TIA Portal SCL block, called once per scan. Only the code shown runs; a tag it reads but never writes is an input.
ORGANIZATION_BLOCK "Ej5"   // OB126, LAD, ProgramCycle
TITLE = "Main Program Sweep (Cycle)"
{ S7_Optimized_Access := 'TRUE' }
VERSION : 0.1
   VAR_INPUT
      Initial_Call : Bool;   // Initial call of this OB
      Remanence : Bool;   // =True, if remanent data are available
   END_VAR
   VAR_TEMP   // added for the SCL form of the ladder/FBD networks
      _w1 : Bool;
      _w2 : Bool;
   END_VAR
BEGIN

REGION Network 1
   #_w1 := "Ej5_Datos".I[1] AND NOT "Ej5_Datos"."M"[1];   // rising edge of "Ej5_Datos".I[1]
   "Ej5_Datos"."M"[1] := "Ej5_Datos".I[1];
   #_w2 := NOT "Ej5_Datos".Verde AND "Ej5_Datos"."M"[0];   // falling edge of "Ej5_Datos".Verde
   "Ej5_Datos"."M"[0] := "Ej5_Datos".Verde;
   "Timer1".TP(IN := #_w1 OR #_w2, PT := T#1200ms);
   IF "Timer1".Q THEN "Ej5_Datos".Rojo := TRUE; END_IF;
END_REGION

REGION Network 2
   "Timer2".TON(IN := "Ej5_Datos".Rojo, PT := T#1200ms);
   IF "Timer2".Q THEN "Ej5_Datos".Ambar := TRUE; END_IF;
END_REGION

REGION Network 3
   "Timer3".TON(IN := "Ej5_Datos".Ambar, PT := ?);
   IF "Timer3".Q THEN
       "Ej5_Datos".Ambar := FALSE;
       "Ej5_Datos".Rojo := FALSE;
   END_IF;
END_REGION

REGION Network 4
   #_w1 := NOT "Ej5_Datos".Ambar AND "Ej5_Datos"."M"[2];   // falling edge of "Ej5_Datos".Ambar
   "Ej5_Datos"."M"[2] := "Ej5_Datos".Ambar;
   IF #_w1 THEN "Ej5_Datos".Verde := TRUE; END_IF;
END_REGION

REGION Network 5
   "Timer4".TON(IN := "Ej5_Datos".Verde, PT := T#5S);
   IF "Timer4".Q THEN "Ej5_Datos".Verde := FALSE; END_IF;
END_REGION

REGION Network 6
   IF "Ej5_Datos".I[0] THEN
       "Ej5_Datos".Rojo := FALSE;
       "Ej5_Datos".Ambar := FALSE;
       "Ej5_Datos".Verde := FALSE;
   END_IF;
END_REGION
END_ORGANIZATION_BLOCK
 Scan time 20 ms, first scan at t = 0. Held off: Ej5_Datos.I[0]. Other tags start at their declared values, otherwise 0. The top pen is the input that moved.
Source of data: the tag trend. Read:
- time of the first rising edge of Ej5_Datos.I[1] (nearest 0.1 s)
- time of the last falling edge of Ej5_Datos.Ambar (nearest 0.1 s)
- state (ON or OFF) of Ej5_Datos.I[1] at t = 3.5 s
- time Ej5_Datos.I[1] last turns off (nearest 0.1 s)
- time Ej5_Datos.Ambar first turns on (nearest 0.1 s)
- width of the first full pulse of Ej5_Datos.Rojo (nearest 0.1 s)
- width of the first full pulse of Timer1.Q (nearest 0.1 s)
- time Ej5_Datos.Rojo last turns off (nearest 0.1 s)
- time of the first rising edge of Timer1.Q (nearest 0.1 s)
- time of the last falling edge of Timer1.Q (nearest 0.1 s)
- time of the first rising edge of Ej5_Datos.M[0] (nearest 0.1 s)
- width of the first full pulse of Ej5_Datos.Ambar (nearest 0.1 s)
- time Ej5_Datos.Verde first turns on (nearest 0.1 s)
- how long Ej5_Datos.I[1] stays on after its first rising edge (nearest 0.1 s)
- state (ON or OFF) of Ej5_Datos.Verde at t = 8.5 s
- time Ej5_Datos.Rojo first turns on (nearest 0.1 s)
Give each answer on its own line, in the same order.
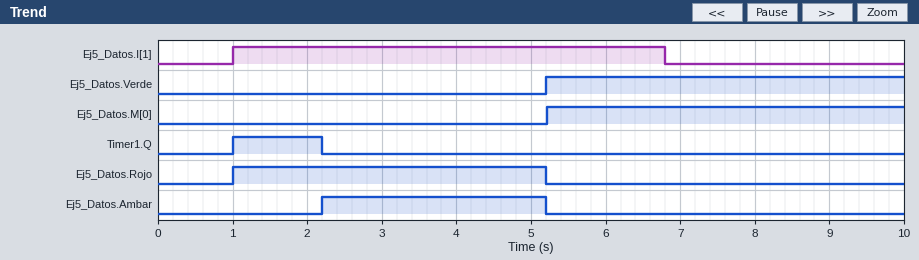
1.0 s
5.2 s
ON
6.8 s
2.2 s
4.2 s
1.2 s
5.2 s
1.0 s
2.2 s
5.2 s
3.0 s
5.2 s
5.8 s
ON
1.0 s
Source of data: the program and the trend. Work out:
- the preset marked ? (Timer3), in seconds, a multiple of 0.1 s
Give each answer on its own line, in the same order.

3.0 s
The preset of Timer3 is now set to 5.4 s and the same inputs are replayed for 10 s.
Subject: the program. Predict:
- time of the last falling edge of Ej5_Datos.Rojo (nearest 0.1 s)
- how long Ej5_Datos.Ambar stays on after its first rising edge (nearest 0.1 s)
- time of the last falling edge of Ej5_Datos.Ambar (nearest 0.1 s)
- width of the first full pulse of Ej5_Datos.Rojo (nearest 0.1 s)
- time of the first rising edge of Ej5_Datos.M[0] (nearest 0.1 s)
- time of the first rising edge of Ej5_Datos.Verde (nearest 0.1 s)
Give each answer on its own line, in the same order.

7.6 s
5.4 s
7.6 s
6.6 s
7.6 s
7.6 s
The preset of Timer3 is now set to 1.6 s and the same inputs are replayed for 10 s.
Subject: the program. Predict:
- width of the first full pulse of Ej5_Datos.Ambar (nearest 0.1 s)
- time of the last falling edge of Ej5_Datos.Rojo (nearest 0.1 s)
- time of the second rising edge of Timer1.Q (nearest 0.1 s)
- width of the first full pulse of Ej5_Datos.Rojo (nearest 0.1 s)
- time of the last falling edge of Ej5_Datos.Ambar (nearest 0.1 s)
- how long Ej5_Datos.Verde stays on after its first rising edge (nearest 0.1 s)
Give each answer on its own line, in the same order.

1.6 s
3.8 s
8.8 s
2.8 s
3.8 s
5.0 s
